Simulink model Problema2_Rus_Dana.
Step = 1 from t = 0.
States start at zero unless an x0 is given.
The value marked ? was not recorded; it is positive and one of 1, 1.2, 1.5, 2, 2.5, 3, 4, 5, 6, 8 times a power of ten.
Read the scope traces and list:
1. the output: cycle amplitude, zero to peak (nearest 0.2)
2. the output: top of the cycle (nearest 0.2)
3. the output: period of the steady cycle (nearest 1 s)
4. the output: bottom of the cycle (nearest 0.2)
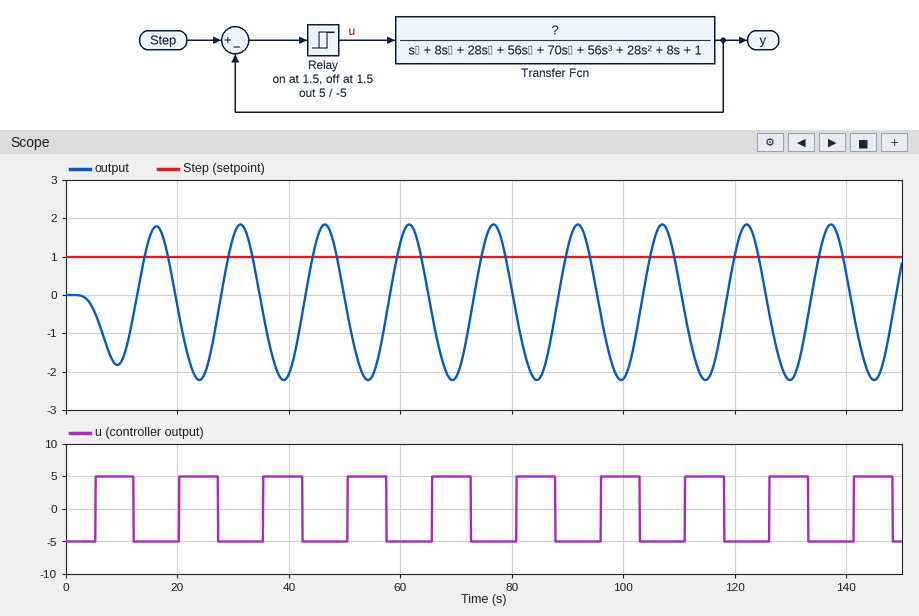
2.0
1.8
15 s
-2.2
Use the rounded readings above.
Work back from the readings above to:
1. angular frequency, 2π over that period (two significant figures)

0.42 rad/s
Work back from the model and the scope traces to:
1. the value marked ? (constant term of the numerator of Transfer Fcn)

0.6
